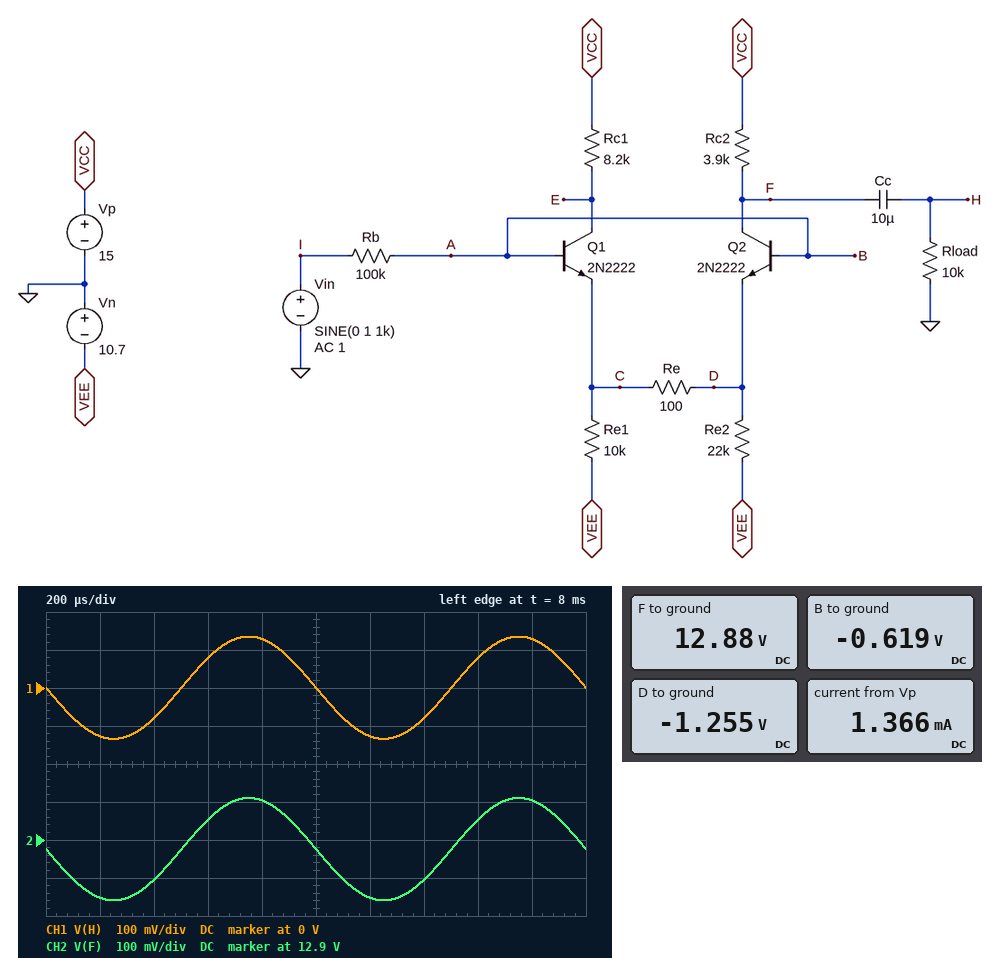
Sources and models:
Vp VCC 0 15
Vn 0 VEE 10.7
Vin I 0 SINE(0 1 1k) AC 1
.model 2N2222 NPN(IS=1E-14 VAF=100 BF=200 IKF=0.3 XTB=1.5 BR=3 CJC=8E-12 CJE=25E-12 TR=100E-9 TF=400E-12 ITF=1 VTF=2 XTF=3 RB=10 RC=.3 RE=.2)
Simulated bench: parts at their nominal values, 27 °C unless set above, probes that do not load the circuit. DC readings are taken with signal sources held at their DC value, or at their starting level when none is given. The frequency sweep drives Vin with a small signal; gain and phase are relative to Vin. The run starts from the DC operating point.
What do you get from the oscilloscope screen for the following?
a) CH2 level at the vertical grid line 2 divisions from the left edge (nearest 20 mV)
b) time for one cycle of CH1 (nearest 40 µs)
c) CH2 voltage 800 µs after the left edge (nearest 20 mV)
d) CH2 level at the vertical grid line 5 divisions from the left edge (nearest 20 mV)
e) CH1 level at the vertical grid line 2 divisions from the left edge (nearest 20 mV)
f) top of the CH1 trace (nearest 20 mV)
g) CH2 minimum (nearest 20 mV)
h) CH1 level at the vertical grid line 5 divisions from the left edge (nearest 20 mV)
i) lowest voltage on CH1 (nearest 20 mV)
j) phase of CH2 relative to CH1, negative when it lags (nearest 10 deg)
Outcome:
12.80 V
1.00 ms
13.00 V
12.88 V
-80 mV
140 mV
12.74 V
0 V
-140 mV
0 deg
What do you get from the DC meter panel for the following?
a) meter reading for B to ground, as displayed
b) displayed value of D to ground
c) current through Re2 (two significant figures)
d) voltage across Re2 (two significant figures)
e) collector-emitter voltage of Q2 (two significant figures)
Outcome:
-0.619 V
-1.255 V
430 µA
9.4 V
14 V
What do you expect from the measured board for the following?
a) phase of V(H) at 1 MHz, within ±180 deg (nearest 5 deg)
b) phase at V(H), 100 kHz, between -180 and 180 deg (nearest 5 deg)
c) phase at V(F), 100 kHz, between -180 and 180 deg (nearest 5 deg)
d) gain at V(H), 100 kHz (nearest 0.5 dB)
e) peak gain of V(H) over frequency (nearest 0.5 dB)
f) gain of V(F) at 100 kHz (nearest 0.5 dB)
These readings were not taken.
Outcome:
85 deg
150 deg
150 deg
-18.5 dB
-17.5 dB
-18.5 dB
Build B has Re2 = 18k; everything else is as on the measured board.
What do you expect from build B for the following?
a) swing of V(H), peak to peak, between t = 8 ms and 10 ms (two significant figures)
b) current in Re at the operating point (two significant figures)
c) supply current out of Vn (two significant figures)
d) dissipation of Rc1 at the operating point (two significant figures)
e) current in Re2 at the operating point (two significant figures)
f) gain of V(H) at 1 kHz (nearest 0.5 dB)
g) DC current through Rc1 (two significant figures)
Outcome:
310 mV
93 µA
1.5 mA
5.8 mW
520 µA
-16.0 dB
840 µA
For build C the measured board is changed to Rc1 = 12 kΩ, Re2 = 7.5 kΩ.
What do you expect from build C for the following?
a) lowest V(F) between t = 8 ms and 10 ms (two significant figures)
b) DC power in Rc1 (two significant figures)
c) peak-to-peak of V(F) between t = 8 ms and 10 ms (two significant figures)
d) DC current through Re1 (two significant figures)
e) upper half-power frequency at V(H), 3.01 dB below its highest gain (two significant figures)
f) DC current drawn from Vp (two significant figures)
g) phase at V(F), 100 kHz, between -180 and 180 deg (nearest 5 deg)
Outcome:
10 V
11 mW
660 mV
910 µA
130 kHz
2.1 mA
140 deg
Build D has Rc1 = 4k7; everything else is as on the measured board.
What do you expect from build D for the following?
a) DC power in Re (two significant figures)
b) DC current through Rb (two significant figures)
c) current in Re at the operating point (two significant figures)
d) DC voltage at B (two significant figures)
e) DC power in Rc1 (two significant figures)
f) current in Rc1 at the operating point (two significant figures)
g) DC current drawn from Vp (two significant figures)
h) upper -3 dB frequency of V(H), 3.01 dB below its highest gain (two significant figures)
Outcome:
1.3 µW
6.1 µA
110 µA
-610 mV
3.2 mW
830 µA
1.4 mA
200 kHz
